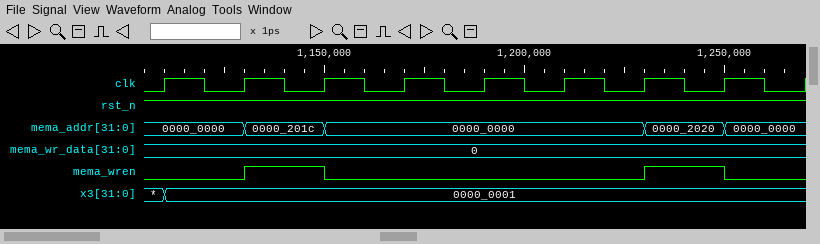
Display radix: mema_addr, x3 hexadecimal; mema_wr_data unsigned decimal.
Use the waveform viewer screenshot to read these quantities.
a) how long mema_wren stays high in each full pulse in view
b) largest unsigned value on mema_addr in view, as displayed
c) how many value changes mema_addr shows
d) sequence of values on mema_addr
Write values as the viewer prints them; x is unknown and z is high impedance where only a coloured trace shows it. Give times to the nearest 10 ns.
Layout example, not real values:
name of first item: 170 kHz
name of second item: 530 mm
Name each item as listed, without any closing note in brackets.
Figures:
how long mema_wren stays high in each full pulse in view: 20 ns, 20 ns
largest unsigned value on mema_addr in view, as displayed: 0000_2020
how many value changes mema_addr shows: 4
sequence of values on mema_addr: 0000_0000, 0000_201c, 0000_0000, 0000_2020, 0000_0000
